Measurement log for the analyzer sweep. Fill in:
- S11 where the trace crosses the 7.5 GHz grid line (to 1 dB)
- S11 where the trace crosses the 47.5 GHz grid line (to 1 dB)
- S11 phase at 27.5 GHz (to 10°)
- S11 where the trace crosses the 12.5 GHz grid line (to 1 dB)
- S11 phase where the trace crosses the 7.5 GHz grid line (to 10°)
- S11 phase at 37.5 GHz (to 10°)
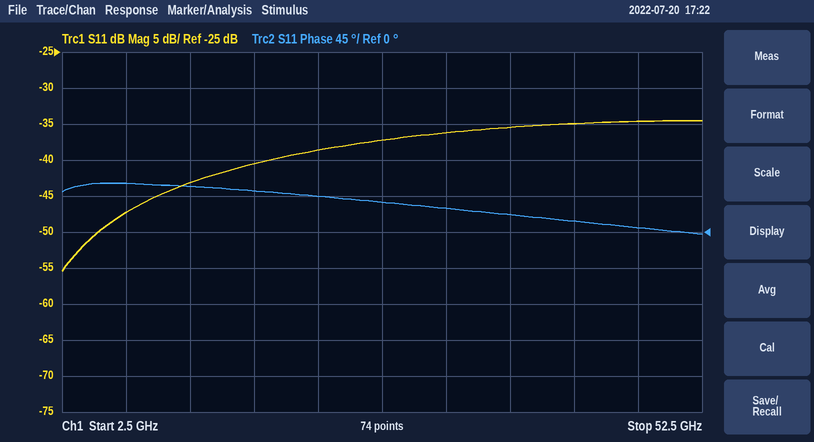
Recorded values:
-47 dB
-35 dB
40°
-43 dB
60°
20°
